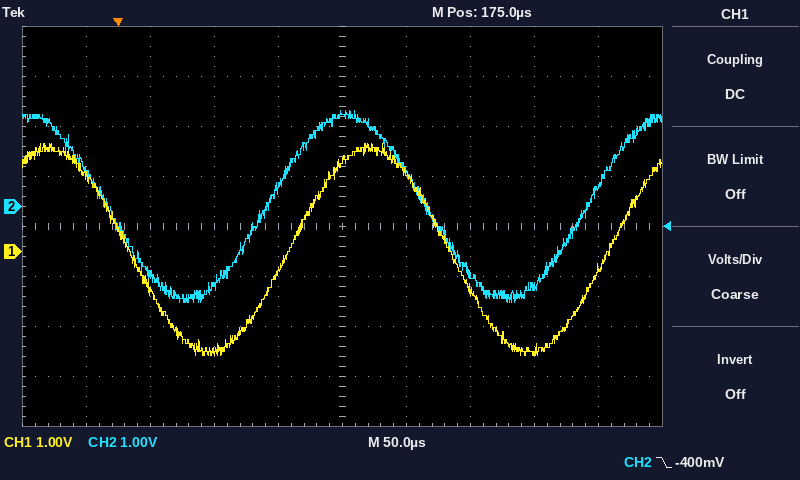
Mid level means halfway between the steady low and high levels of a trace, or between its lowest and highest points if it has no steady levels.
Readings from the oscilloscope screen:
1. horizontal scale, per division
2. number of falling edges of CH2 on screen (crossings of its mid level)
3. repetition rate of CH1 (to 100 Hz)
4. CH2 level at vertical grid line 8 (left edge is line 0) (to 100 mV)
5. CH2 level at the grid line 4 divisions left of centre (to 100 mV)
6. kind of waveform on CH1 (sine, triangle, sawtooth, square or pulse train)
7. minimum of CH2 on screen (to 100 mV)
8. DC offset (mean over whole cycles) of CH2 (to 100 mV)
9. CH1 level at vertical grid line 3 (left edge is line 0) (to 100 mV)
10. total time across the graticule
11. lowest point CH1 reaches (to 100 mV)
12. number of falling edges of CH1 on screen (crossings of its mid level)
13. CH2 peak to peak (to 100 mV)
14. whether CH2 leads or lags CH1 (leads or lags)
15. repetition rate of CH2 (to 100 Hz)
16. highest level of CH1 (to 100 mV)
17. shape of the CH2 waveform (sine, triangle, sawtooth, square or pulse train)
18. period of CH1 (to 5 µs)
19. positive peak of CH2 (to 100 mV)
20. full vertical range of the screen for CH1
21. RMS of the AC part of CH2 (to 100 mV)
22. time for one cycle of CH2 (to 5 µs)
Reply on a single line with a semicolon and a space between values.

50 µs; 2; 4.0 kHz; -1.6 V; 700 mV; sine; -1.9 V; 0.0 V; -2.0 V; 500 µs; -2.1 V; 2; 3.8 V; leads; 4.0 kHz; 2.2 V; sine; 250 µs; 1.9 V; 8 V; 1.3 V; 250 µs
